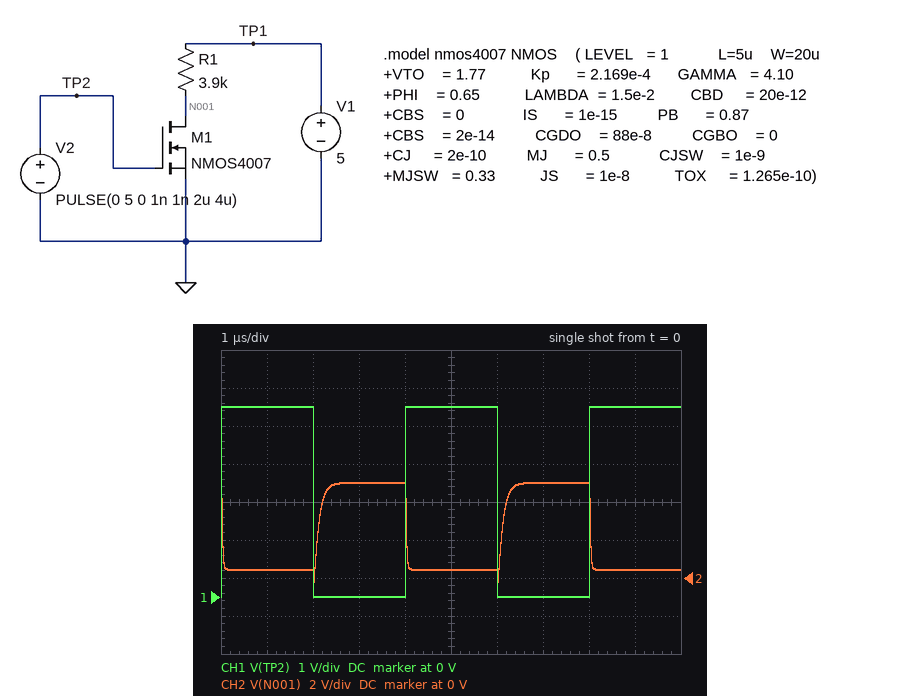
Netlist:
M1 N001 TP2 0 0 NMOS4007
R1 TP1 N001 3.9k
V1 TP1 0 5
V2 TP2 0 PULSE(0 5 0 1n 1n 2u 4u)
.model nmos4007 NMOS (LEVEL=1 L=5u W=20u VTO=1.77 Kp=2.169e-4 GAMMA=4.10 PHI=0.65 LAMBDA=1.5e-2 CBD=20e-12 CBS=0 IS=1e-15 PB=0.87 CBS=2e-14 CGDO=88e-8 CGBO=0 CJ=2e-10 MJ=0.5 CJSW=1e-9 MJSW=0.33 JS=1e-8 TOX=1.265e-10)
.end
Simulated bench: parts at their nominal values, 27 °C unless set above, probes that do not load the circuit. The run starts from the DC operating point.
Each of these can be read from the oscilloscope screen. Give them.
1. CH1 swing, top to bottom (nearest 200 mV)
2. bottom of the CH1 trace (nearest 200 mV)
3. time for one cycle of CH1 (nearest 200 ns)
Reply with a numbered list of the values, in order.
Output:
1. 5.0 V
2. 0 V
3. 4.0 µs
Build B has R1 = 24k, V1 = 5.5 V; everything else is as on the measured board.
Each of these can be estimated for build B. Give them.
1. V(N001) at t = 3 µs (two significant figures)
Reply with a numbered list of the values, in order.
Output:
1. 3.9 V
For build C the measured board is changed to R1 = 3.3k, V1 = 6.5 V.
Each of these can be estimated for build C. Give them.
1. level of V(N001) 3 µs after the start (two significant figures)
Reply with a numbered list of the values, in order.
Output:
1. 6.5 V
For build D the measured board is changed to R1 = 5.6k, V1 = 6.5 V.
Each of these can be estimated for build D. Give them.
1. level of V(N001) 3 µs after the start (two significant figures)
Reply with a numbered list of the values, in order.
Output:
1. 6.5 V
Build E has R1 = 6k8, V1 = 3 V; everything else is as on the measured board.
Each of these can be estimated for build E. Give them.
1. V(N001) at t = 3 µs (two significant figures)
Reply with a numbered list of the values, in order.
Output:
1. 3.0 V
